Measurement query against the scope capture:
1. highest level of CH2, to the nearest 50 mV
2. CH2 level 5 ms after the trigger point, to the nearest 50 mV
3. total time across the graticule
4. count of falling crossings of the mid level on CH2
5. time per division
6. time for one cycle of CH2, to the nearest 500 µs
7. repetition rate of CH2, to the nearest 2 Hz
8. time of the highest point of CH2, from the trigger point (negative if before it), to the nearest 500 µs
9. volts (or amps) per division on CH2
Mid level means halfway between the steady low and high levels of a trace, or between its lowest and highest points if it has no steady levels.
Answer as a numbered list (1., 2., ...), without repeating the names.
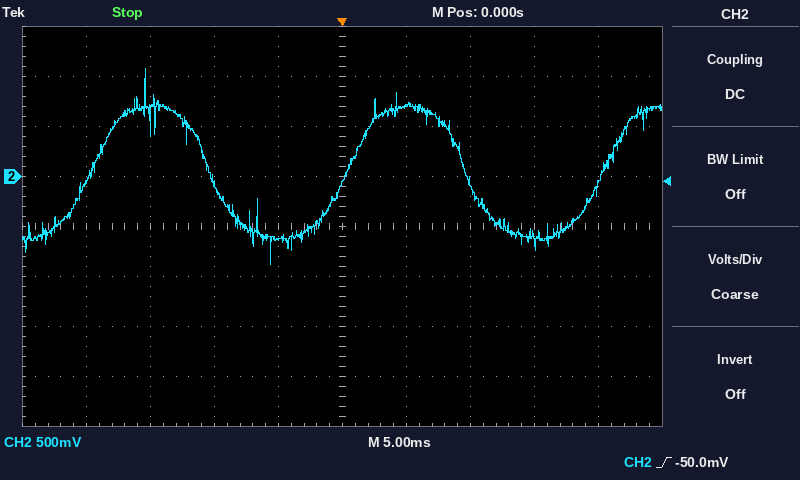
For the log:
1. 1.10 V
2. 700 mV
3. 50 ms
4. 2
5. 5 ms
6. 20.0 ms
7. 50 Hz
8. -15.5 ms
9. 500 mV
